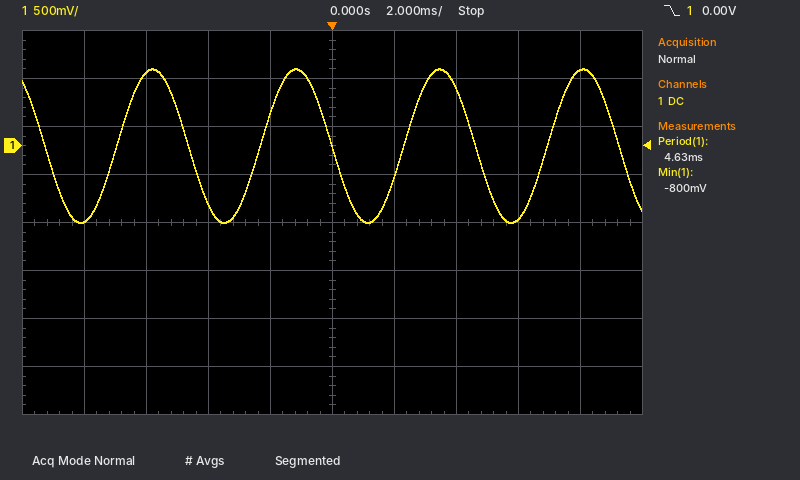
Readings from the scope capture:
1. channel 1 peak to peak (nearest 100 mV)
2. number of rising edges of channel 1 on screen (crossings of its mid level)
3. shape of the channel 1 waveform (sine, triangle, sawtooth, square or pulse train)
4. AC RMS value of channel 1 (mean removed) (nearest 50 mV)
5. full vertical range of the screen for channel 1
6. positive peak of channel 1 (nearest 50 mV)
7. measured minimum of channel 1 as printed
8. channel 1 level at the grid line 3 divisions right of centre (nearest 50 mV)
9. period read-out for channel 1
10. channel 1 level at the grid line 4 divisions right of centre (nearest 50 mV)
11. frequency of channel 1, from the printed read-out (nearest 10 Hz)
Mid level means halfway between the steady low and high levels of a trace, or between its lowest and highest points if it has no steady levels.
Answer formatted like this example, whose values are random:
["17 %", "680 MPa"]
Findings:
["1.60 V", "4", "sine", "550 mV", "4 V", "800 mV", "-800 mV", "-750 mV", "4.63 ms", "800 mV", "220 Hz"]
